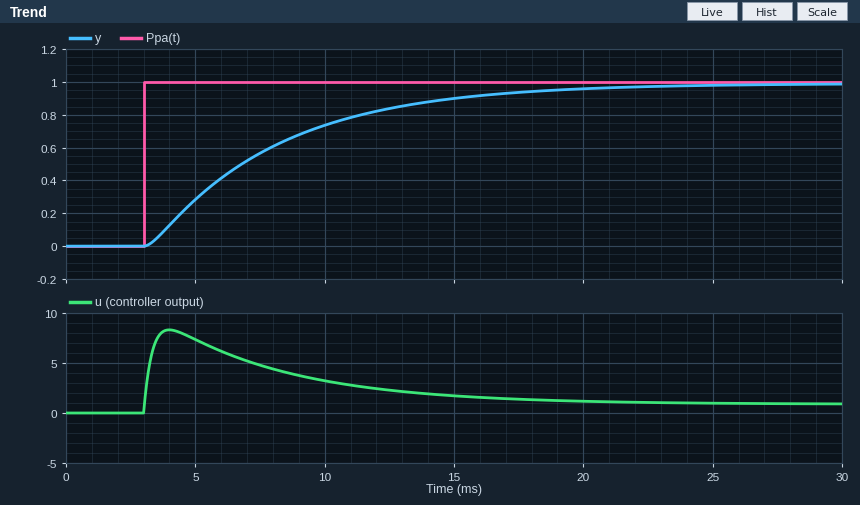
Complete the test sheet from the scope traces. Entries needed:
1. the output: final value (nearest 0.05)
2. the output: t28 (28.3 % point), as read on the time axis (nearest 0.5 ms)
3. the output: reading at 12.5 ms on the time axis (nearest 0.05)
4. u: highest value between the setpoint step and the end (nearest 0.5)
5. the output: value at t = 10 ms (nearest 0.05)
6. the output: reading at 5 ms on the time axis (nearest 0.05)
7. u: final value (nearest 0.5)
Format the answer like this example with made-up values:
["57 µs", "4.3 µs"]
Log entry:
["1.00", "5.0 ms", "0.85", "8.5", "0.75", "0.30", "1.0"]
